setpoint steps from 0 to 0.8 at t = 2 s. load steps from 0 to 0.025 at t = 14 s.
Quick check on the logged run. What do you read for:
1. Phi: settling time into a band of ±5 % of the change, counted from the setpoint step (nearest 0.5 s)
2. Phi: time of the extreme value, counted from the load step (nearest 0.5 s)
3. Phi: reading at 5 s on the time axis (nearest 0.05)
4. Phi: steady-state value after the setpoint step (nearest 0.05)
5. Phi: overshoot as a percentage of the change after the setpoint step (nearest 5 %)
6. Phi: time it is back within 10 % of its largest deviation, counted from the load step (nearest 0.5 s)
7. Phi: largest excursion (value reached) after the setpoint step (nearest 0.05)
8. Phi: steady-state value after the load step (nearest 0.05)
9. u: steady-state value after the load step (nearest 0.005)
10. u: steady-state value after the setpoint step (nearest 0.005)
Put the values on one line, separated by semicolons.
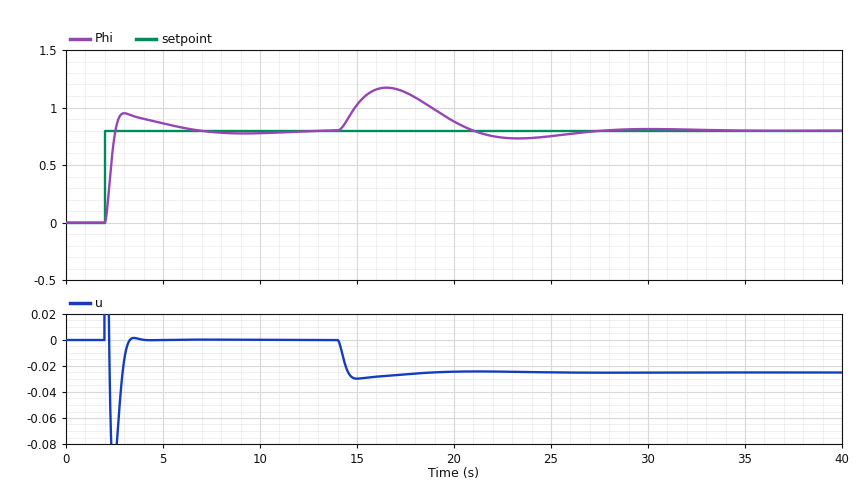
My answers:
3.5 s; 2.5 s; 0.85; 0.80; 20 %; 11.5 s; 0.95; 0.80; -0.025; 0.000
